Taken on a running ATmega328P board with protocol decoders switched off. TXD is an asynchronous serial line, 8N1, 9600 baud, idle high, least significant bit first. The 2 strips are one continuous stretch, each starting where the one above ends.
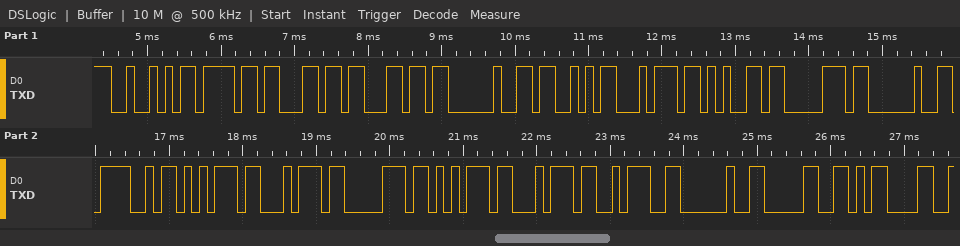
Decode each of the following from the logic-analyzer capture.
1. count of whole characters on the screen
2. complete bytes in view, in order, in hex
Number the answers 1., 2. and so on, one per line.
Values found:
1. 20
2. 52 6F 6C 6C 20 53 74 65 70 20 4F 75 74 70 75 74 3A 20 30 0D
